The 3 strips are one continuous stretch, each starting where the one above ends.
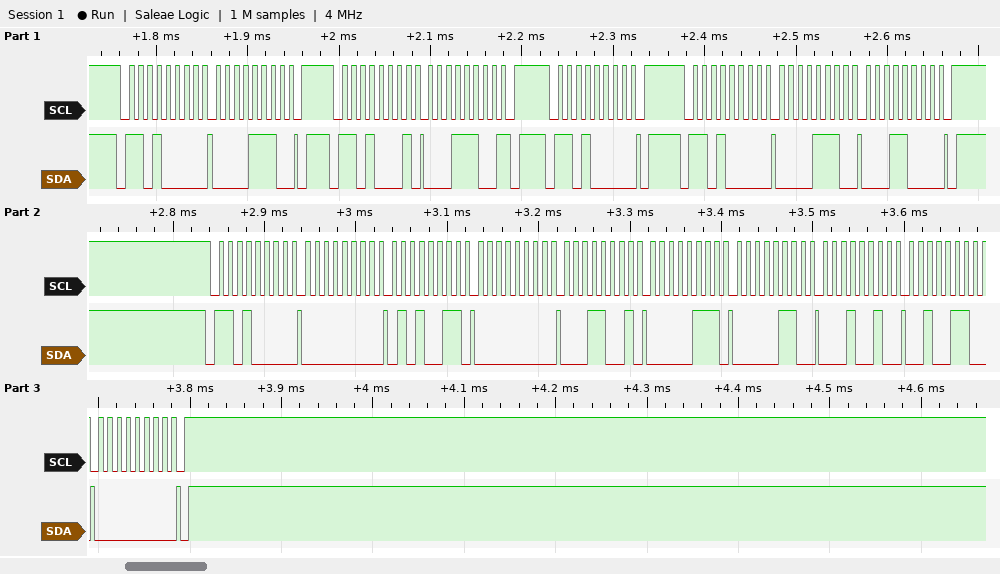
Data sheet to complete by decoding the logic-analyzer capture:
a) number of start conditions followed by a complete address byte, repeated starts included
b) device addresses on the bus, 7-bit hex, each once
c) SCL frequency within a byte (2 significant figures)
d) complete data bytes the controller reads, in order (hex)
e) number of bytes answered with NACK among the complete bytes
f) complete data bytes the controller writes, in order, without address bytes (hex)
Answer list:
5
0x68
100 kHz
1C
1
0E 0E 18 00 53 00 19 07 06 12 26 00
